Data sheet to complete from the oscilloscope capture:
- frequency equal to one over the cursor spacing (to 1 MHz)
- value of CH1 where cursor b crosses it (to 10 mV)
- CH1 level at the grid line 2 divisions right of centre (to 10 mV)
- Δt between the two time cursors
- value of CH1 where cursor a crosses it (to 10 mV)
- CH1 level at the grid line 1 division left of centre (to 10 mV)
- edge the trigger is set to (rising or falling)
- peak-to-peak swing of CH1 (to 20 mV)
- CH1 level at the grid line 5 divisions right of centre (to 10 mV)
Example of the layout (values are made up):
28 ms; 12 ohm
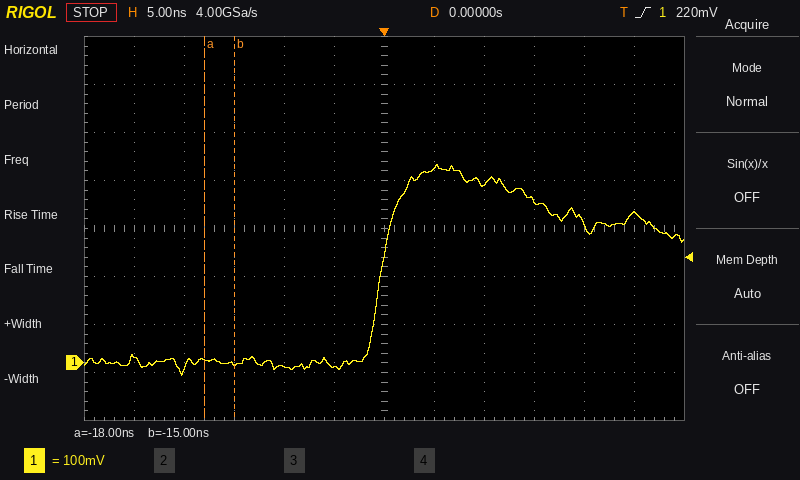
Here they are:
333 MHz; 0 mV; 370 mV; 3.0 ns; 10 mV; -10 mV; rising; 440 mV; 310 mV
